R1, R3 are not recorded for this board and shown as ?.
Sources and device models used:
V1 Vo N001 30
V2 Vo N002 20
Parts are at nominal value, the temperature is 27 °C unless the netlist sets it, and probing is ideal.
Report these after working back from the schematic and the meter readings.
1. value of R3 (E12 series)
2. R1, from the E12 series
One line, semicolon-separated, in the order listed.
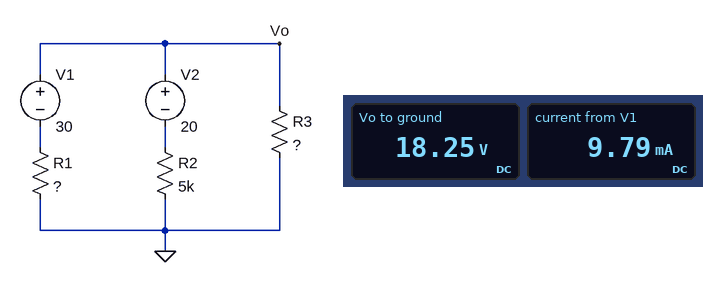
1.8 kΩ; 1.2 kΩ
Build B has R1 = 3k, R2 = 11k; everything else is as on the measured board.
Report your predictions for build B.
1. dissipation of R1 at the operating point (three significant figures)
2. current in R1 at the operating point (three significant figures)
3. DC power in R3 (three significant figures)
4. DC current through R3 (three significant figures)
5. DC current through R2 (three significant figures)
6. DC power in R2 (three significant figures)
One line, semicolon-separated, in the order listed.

107 mW; 5.98 mA; 80.8 mW; 6.70 mA; 722 µA; 5.73 mW
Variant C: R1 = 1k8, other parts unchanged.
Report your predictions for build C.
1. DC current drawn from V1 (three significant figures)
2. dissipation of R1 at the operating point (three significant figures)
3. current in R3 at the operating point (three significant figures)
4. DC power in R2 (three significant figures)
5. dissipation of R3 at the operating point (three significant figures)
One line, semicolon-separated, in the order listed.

7.91 mA; 113 mW; 8.76 mA; 3.59 mW; 138 mW
